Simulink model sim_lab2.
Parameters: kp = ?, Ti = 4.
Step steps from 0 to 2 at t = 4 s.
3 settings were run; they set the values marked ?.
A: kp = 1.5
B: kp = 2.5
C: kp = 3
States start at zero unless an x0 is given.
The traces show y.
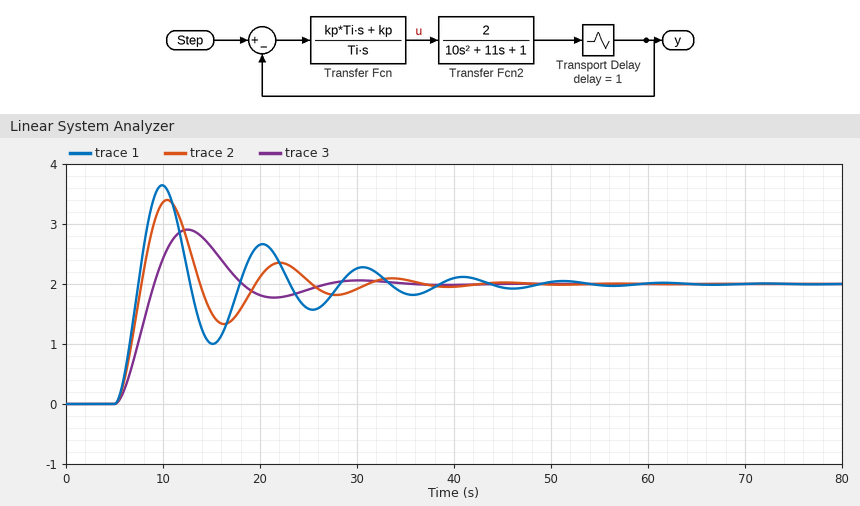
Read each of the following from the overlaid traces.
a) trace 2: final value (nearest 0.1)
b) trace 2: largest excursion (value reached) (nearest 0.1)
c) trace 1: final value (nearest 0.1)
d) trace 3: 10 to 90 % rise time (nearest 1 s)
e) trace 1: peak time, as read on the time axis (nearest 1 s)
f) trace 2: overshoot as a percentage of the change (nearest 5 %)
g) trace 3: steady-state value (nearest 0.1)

2.0
3.4
2.0
3 s
10 s
70 %
2.0
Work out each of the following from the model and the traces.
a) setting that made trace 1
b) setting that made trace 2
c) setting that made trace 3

C
B
A
